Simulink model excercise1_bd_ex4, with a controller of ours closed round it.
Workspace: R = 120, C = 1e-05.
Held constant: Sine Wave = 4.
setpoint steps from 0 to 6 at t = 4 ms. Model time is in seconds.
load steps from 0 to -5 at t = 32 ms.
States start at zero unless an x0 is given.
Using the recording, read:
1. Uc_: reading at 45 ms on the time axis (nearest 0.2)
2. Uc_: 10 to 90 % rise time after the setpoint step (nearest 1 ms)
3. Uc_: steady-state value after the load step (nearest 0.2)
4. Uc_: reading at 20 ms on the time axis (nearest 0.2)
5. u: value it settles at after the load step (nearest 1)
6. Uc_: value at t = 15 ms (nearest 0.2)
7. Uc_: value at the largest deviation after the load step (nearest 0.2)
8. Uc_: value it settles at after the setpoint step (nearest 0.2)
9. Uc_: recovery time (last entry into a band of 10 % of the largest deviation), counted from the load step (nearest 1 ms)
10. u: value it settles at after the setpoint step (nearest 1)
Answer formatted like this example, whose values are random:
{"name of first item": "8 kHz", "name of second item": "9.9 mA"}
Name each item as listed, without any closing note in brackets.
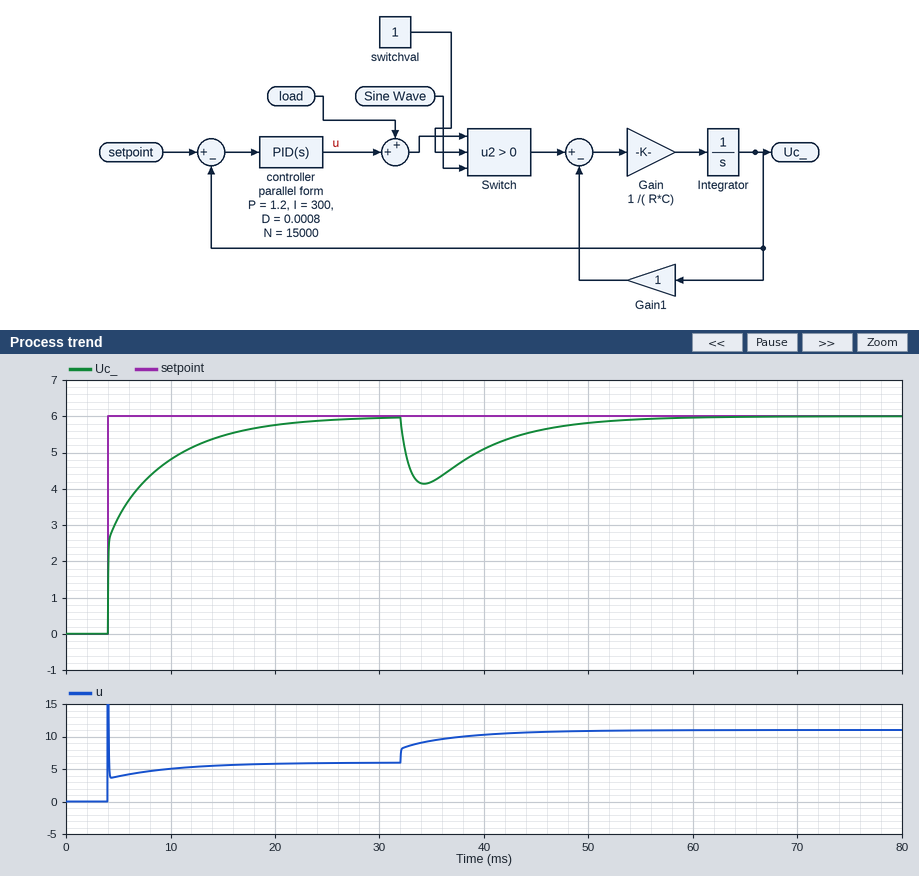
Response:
{"Uc_: reading at 45 ms on the time axis": "5.6", "Uc_: 10 to 90 % rise time after the setpoint step": "10 ms", "Uc_: steady-state value after the load step": "6.0", "Uc_: reading at 20 ms on the time axis": "5.8", "u: value it settles at after the load step": "11", "Uc_: value at t = 15 ms": "5.4", "Uc_: value at the largest deviation after the load step": "4.2", "Uc_: value it settles at after the setpoint step": "6.0", "Uc_: recovery time (last entry into a band of 10 % of the largest deviation), counted from the load step": "18 ms", "u: value it settles at after the setpoint step": "6"}
